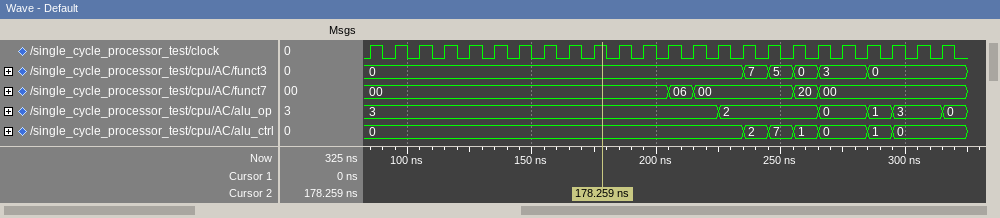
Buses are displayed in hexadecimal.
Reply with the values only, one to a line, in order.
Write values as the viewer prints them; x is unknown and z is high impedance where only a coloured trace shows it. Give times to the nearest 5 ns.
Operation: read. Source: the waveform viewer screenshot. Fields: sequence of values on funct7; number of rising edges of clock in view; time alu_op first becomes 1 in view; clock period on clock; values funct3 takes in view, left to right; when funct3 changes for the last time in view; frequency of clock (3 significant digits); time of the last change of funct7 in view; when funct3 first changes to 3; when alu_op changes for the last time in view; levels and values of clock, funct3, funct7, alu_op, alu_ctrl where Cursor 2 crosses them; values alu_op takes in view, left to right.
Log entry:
00, 06, 00, 20, 00
24
285 ns
10 ns
0, 7, 5, 0, 3, 0
285 ns
100 MHz
265 ns
265 ns
315 ns
clock=1, funct3=0, funct7=00, alu_op=3, alu_ctrl=0
3, 2, 0, 1, 3, 0
